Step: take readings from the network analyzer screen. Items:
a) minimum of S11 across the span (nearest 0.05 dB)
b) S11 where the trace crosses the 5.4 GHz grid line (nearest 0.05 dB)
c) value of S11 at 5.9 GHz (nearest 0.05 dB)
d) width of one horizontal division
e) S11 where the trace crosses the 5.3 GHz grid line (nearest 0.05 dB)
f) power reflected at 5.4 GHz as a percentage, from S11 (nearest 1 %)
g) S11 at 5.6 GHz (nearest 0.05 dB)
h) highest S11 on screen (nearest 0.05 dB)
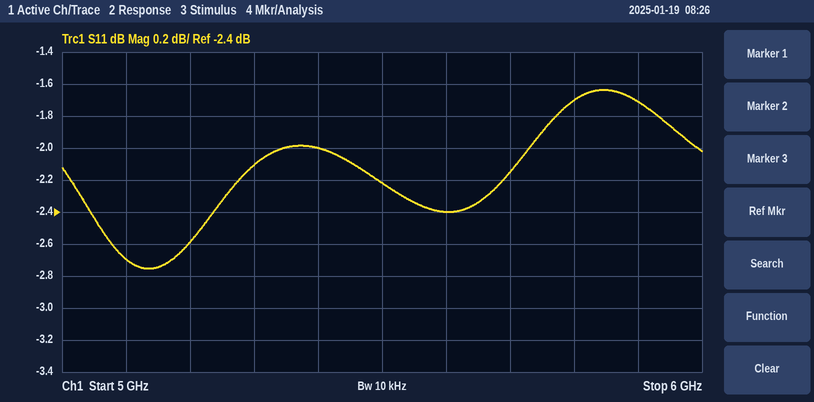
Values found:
-2.75 dB
-2.00 dB
-1.70 dB
100 MHz
-2.10 dB
63 %
-2.40 dB
-1.65 dB
